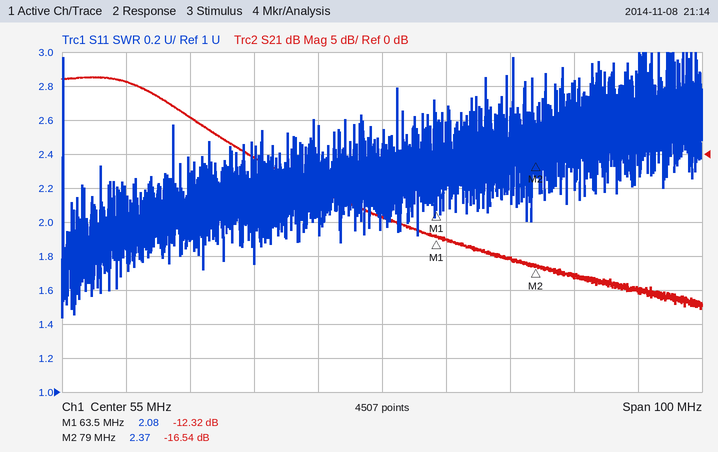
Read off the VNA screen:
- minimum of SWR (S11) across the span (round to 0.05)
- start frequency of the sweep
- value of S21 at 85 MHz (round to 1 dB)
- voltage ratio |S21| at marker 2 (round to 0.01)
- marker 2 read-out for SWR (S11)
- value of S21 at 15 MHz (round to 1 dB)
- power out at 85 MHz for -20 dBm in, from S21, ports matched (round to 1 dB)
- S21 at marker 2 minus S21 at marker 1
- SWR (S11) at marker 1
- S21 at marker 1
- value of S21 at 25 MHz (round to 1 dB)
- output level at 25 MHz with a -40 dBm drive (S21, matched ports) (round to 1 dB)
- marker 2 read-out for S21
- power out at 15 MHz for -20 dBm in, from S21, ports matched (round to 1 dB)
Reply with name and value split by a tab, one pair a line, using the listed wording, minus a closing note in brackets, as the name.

minimum of SWR (S11) across the span	1.45
start frequency of the sweep	5 MHz
value of S21 at 85 MHz	-18 dB
voltage ratio |S21| at marker 2	0.15
marker 2 read-out for SWR	2.37
value of S21 at 15 MHz	11 dB
power out at 85 MHz for -20 dBm in, from S21, ports matched	-38 dBm
S21 at marker 2 minus S21 at marker 1	-4.22 dB
SWR (S11) at marker 1	2.08
S21 at marker 1	-12.32 dB
value of S21 at 25 MHz	5 dB
output level at 25 MHz with a -40 dBm drive (S21, matched ports)	-35 dBm
marker 2 read-out for S21	-16.54 dB
power out at 15 MHz for -20 dBm in, from S21, ports matched	-9 dBm
